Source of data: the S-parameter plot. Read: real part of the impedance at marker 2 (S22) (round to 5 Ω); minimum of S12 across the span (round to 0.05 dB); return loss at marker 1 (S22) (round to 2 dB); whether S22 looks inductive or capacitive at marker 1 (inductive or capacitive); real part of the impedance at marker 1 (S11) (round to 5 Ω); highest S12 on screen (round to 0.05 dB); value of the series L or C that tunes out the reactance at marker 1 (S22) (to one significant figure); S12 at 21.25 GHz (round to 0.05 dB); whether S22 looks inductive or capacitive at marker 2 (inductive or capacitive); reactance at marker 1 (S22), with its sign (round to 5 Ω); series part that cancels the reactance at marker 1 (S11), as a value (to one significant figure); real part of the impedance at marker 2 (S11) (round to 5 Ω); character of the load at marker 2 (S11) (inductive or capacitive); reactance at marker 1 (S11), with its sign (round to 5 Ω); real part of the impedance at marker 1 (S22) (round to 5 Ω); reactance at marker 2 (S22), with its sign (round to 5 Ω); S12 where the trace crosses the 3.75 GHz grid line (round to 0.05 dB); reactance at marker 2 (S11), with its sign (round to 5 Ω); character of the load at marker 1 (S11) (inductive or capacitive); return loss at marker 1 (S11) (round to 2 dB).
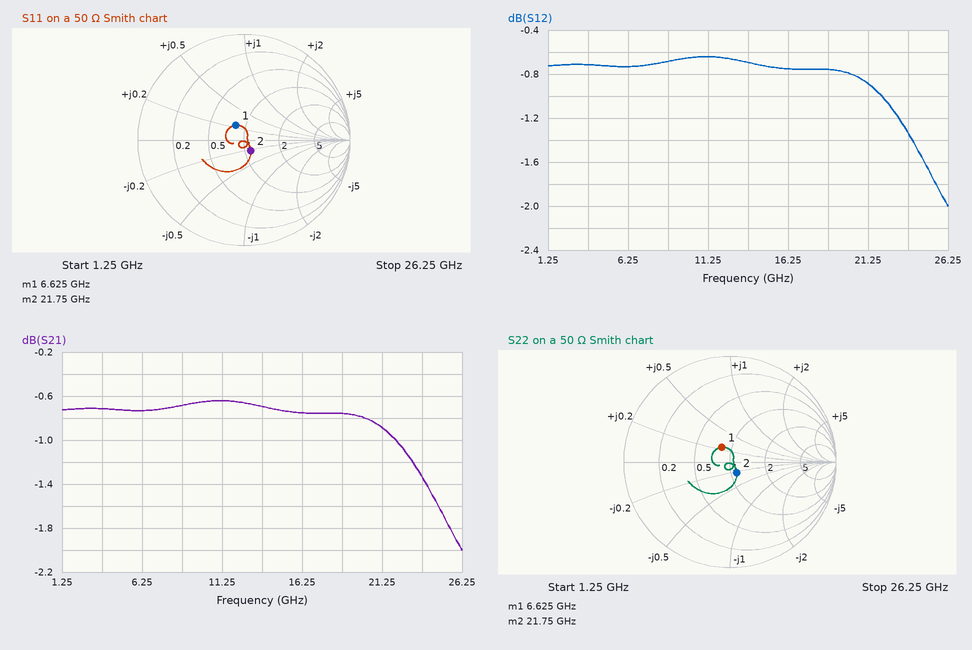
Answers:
55 Ω
-2.00 dB
16 dB
inductive
40 Ω
-0.65 dB
2 pF
-0.90 dB
capacitive
+10 Ω
2 pF
55 Ω
capacitive
+10 Ω
40 Ω
-10 Ω
-0.70 dB
-10 Ω
inductive
16 dB
